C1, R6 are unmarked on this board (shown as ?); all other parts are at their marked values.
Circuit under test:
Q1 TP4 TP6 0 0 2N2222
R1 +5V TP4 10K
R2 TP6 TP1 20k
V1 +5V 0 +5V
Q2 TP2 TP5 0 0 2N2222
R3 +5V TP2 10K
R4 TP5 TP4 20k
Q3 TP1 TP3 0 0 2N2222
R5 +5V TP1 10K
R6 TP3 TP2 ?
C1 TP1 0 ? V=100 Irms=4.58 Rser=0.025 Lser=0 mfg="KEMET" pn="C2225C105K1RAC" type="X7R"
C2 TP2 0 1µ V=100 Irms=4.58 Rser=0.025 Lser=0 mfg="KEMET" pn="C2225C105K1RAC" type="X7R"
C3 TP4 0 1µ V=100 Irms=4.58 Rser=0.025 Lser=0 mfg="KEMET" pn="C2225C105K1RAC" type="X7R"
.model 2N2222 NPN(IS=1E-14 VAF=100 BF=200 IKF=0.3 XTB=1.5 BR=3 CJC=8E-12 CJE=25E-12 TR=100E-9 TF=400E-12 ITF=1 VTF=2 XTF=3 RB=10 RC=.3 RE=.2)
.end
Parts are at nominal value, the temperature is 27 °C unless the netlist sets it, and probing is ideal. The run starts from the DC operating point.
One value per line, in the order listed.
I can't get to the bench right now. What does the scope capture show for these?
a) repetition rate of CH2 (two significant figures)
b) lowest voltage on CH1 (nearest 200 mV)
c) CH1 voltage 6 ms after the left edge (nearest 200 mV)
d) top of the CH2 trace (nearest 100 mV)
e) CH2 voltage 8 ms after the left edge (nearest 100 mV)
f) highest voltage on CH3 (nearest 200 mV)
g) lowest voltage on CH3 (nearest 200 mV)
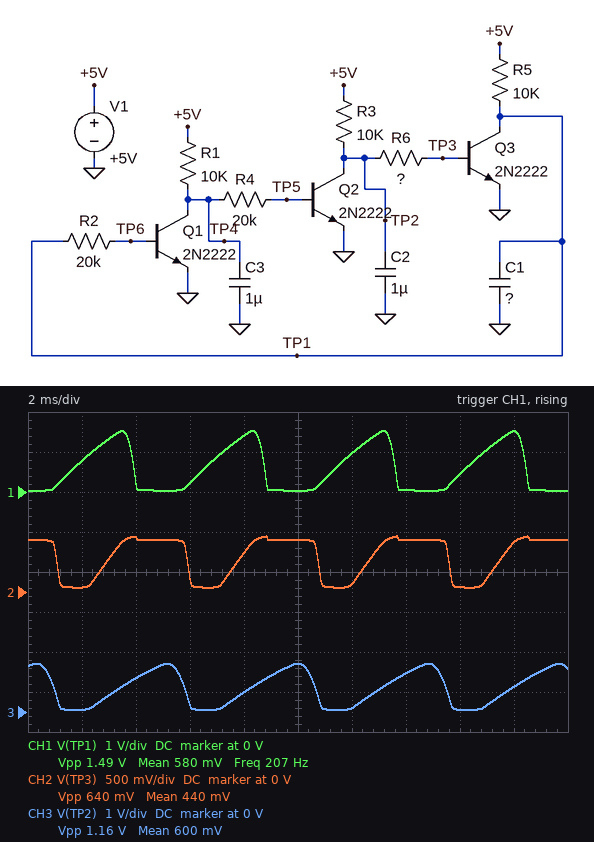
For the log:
210 Hz
0 V
200 mV
700 mV
500 mV
1.2 V
0 V
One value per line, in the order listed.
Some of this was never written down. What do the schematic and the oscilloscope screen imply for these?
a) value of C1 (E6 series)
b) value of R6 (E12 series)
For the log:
680 nF
6.8 kΩ
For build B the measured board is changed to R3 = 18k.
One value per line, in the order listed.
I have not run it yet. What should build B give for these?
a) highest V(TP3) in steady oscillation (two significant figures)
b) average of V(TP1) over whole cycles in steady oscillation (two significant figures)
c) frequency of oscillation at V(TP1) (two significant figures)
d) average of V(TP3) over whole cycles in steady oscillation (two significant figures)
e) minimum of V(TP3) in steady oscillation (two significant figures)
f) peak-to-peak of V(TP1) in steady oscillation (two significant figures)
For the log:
690 mV
870 mV
170 Hz
420 mV
43 mV
1.9 V
